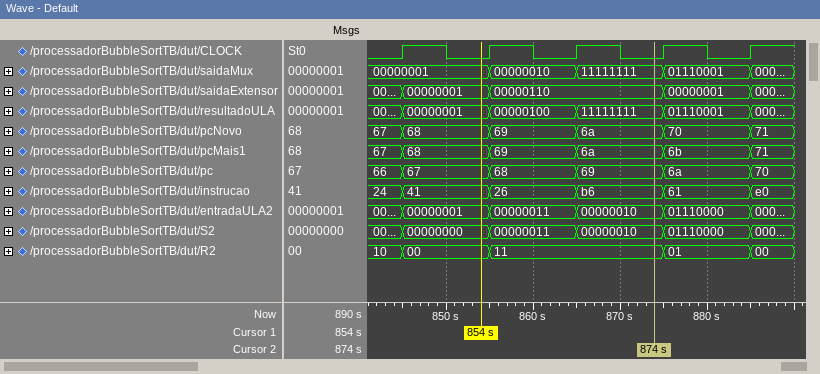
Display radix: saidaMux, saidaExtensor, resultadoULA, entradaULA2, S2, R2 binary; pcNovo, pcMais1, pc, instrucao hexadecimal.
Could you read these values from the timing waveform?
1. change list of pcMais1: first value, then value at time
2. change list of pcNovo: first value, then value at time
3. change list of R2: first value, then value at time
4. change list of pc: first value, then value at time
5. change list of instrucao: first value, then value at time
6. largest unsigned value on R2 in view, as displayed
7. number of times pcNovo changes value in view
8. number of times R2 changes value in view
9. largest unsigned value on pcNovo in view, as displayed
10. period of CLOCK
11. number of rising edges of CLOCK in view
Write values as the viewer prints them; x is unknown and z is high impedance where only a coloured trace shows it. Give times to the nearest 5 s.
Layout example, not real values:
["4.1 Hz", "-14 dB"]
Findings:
["67, 68 at 845 s, 69 at 855 s, 6a at 865 s, 6b at 875 s, 71 at 885 s", "67, 68 at 845 s, 69 at 855 s, 6a at 865 s, 70 at 875 s, 71 at 885 s", "10, 00 at 845 s, 11 at 855 s, 01 at 875 s, 00 at 885 s", "66, 67 at 845 s, 68 at 855 s, 69 at 865 s, 6a at 875 s, 70 at 885 s", "24, 41 at 845 s, 26 at 855 s, b6 at 865 s, 61 at 875 s, e0 at 885 s", "11", "5", "4", "71", "10 s", "5"]
